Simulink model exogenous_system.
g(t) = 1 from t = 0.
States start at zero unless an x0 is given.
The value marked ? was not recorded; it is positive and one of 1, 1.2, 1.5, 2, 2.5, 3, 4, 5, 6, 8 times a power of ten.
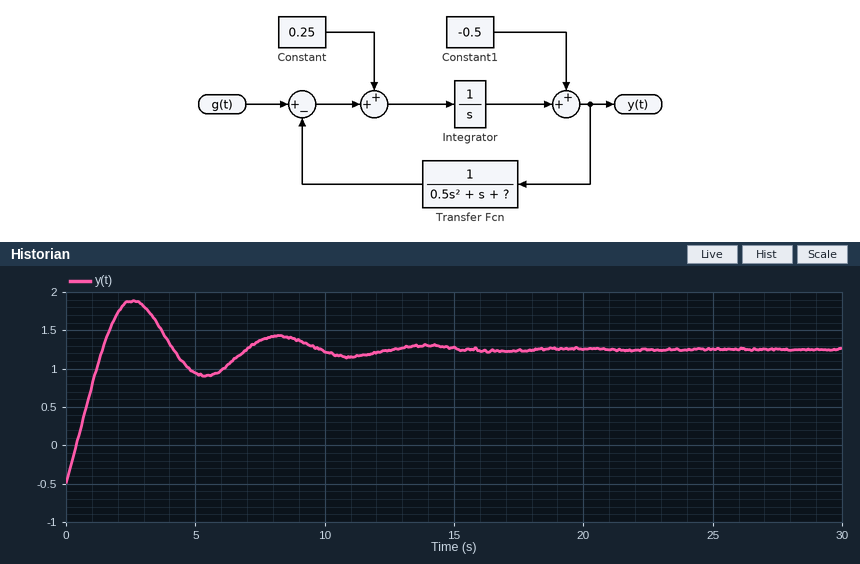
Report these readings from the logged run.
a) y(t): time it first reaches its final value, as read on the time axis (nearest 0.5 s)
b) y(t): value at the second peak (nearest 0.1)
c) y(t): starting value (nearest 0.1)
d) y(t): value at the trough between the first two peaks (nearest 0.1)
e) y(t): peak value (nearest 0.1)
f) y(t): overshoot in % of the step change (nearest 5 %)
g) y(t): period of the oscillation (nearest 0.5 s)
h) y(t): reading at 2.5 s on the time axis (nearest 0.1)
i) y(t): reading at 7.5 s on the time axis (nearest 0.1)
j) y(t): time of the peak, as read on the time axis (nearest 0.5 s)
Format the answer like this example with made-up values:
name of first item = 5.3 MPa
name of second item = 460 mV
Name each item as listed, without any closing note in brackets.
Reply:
y(t): time it first reaches its final value, as read on the time axis = 1.5 s
y(t): value at the second peak = 1.4
y(t): starting value = -0.5
y(t): value at the trough between the first two peaks = 0.9
y(t): peak value = 1.9
y(t): overshoot in % of the step change = 35 %
y(t): period of the oscillation = 5.5 s
y(t): reading at 2.5 s on the time axis = 1.9
y(t): reading at 7.5 s on the time axis = 1.4
y(t): time of the peak, as read on the time axis = 2.5 s
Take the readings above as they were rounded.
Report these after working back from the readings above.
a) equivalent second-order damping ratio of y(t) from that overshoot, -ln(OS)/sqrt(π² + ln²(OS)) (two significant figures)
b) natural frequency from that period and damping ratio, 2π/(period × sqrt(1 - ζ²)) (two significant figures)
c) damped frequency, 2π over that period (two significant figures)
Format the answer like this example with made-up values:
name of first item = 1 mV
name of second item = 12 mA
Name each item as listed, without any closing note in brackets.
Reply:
equivalent second-order damping ratio of y(t) from that overshoot, -ln(OS)/sqrt(π² + ln²(OS)) = 0.32
natural frequency from that period and damping ratio, 2π/(period × sqrt(1 - ζ²)) = 1.2 rad/s
damped frequency, 2π over that period = 1.1 rad/s
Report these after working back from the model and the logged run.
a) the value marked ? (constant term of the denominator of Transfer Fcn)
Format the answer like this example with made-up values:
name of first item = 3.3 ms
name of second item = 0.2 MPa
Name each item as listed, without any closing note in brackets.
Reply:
the value marked ? = 1
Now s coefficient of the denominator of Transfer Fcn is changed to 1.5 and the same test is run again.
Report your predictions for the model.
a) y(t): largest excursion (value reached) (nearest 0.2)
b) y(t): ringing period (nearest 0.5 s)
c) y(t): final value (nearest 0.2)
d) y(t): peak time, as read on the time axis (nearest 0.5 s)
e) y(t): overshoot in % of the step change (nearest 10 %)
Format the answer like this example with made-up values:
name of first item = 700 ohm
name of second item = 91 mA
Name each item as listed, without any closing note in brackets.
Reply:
y(t): largest excursion (value reached) = 2.0
y(t): ringing period = 7.5 s
y(t): final value = 1.2
y(t): peak time, as read on the time axis = 3.0 s
y(t): overshoot in % of the step change = 50 %
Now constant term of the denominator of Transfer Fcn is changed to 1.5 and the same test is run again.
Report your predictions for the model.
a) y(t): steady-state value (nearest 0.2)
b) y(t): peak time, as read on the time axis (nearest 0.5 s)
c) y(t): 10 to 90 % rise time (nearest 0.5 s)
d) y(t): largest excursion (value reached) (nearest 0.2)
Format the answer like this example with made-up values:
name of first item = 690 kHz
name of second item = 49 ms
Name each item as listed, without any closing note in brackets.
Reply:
y(t): steady-state value = 1.8
y(t): peak time, as read on the time axis = 3.0 s
y(t): 10 to 90 % rise time = 1.5 s
y(t): largest excursion (value reached) = 2.0
